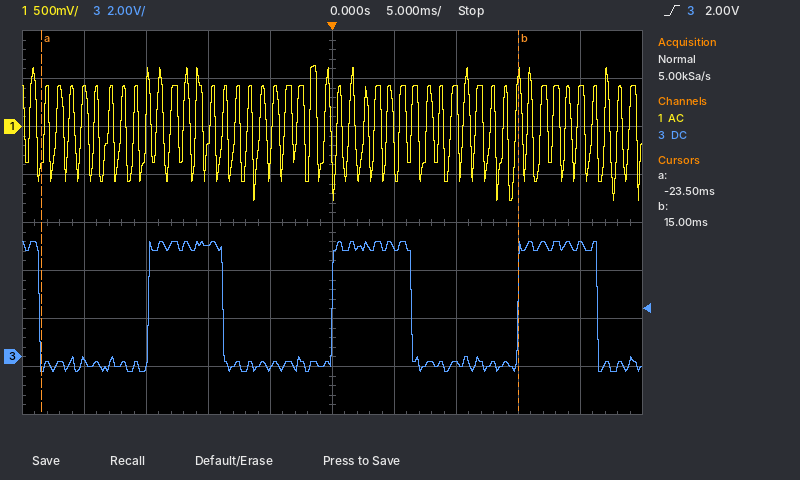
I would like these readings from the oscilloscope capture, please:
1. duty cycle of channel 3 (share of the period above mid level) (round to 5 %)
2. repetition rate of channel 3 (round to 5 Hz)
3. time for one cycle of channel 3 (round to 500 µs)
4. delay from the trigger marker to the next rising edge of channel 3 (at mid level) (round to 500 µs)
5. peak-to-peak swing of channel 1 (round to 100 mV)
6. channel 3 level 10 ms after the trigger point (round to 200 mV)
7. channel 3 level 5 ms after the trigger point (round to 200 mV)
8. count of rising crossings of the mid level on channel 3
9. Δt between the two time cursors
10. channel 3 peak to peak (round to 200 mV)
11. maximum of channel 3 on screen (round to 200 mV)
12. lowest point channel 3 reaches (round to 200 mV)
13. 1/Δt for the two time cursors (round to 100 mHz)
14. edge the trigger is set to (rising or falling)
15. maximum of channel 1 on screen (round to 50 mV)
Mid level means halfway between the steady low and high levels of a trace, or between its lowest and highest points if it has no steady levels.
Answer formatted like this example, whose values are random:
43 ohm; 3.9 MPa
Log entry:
40 %; 65 Hz; 15.0 ms; 15.0 ms; 1.40 V; -200 mV; 4.6 V; 3; 38.5 ms; 5.4 V; 4.8 V; -600 mV; 26.0 Hz; rising; 650 mV
